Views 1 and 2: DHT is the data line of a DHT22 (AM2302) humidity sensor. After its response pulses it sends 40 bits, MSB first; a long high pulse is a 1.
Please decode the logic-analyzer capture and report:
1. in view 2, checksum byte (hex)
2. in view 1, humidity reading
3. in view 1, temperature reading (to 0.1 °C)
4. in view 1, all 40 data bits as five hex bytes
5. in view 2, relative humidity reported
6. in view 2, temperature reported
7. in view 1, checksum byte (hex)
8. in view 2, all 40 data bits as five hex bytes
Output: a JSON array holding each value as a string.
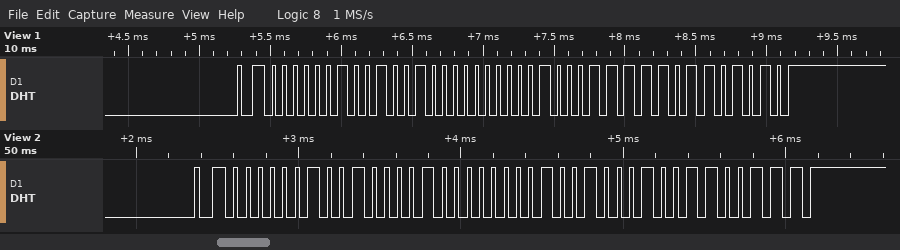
["0x67", "58.4 %", "28.7 °C", "02 48 01 1F 6A", "57.8 %", "29.0 °C", "0x6A", "02 42 01 22 67"]
